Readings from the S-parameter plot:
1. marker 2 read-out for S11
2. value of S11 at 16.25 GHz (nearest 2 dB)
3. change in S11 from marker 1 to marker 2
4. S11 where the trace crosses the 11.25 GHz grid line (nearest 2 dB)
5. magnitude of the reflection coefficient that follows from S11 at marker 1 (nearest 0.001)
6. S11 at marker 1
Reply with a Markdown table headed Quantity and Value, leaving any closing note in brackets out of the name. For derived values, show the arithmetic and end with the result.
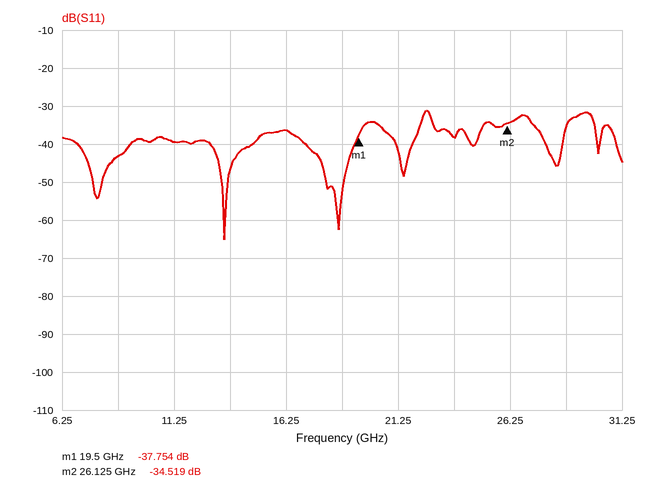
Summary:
| Quantity | Value |
|---|---|
| marker 2 read-out for S11 | -34.519 dB |
| value of S11 at 16.25 GHz | -36 dB |
| change in S11 from marker 1 to marker 2 | -34.519 − (-37.754) = 3.235 dB |
| S11 where the trace crosses the 11.25 GHz grid line | -40 dB |
| magnitude of the reflection coefficient that follows from S11 at marker 1 | 10^(-37.754/20) ≈ 0.013 |
| S11 at marker 1 | -37.754 dB |
